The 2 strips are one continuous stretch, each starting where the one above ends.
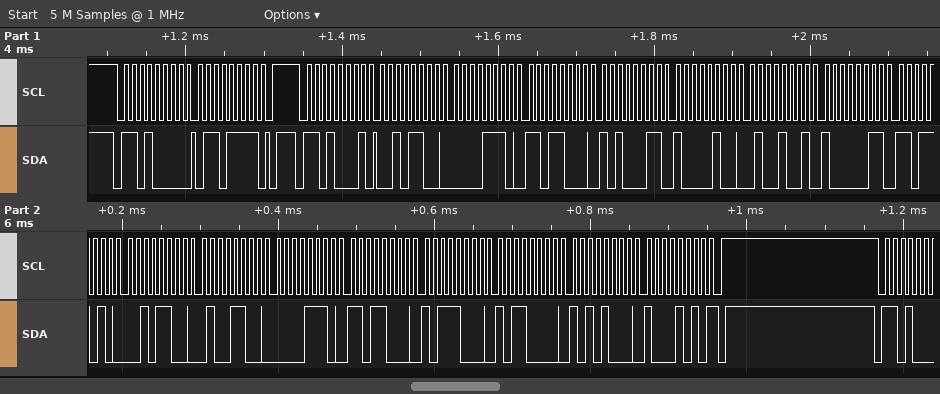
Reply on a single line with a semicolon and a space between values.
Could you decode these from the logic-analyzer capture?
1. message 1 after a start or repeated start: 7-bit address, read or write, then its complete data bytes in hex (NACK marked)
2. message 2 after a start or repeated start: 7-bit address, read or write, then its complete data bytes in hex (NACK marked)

0x68 write: 6F; 0x68 read: 2C 0E D8 A3 84 49 83 DA 2C 4C 0E D8 B8 B0 A8 8A NACK
